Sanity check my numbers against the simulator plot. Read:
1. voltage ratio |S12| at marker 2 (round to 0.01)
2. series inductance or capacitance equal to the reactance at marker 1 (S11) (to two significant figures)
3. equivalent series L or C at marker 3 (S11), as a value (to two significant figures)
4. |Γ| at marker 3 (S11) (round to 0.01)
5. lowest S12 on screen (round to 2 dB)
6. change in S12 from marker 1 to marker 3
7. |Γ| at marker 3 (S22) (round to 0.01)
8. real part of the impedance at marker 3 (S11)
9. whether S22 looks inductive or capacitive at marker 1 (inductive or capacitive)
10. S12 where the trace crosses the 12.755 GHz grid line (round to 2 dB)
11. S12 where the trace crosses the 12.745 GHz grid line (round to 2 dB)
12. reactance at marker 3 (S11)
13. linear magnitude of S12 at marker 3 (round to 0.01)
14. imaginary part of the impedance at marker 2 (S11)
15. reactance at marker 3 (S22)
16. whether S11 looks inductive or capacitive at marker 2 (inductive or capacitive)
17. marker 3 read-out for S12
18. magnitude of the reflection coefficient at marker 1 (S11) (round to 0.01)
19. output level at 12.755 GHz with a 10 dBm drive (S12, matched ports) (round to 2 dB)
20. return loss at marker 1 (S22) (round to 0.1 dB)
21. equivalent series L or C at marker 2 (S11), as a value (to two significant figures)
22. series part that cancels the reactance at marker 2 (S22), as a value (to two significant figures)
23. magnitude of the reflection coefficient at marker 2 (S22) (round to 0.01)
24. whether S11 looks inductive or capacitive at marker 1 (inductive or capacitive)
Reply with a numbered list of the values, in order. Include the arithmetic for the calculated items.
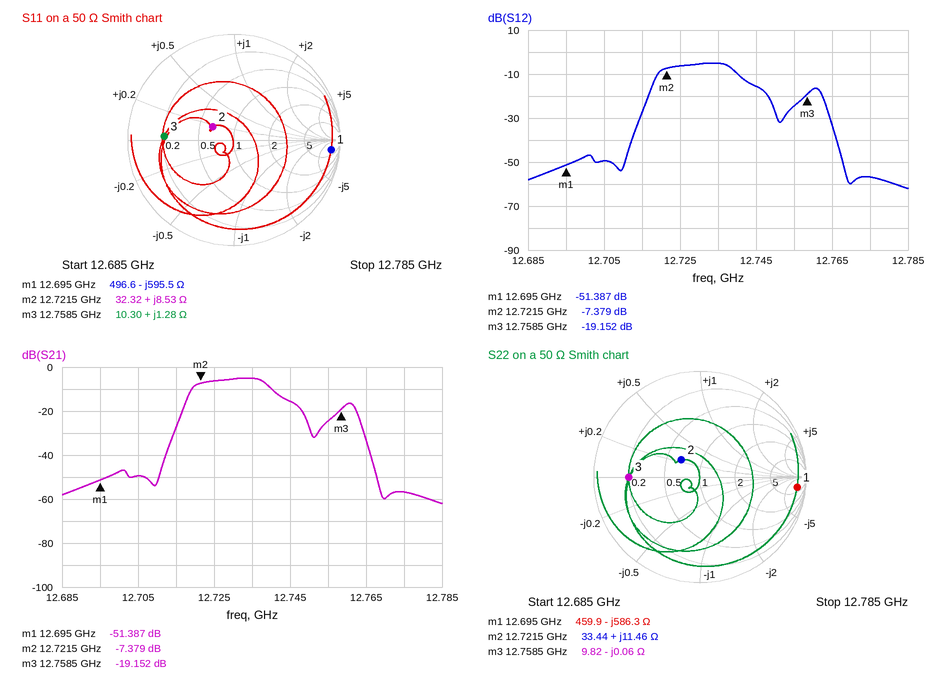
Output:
1. 10^(-7.379/20) ≈ 0.43
2. C = 1/(2π × 12.695 GHz × 595.5 Ω) ≈ 21 fF
3. L = 1.28 Ω/(2π × 12.7585 GHz) ≈ 16 pH
4. 0.66
5. -62 dB
6. -19.152 − (-51.387) = 32.235 dB
7. 0.67
8. 10.30 Ω
9. capacitive
10. -24 dB
11. -16 dB
12. +1.28 Ω
13. 10^(-19.152/20) ≈ 0.11
14. +8.53 Ω
15. -0.06 Ω
16. inductive
17. -19.152 dB
18. 0.92
19. 10 dBm + (-24 dB) = -14 dBm
20. 0.7 dB
21. L = 8.53 Ω/(2π × 12.7215 GHz) ≈ 107 pH, so 110 pH to two significant figures
22. C = 1/(2π × 12.7215 GHz × 11.46 Ω) ≈ 1.1 pF
23. 0.24
24. capacitive
